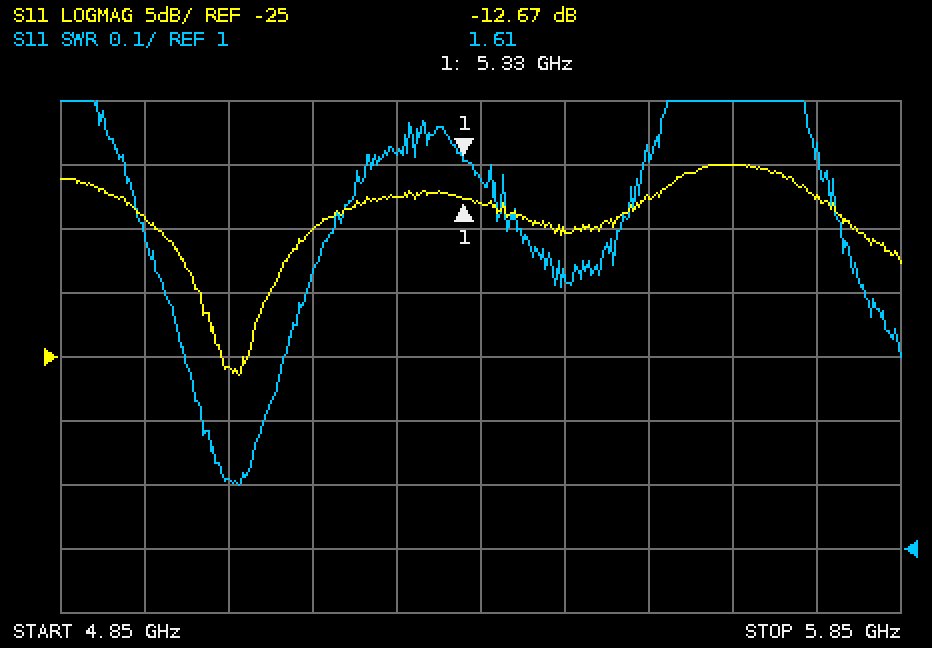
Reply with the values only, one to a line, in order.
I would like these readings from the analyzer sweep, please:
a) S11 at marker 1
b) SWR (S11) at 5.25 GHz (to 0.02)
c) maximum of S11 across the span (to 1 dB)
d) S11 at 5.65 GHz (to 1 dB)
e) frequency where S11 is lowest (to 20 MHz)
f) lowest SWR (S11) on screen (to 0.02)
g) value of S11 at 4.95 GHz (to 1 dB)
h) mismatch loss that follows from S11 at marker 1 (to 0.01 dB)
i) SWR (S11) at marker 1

-12.67 dB
1.62
-10 dB
-10 dB
5.06 GHz
1.10
-14 dB
0.24 dB
1.61
